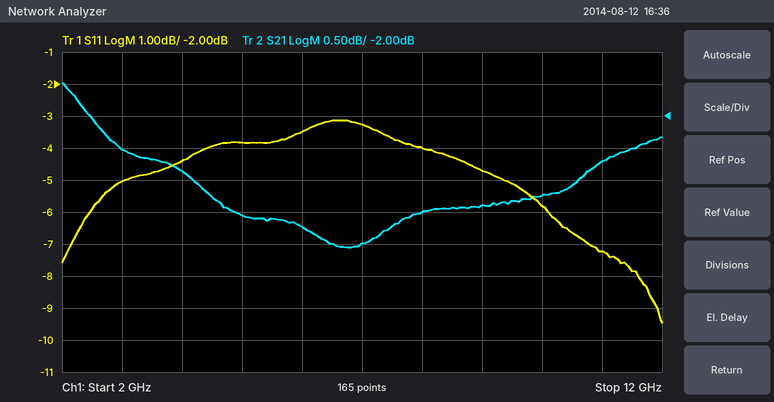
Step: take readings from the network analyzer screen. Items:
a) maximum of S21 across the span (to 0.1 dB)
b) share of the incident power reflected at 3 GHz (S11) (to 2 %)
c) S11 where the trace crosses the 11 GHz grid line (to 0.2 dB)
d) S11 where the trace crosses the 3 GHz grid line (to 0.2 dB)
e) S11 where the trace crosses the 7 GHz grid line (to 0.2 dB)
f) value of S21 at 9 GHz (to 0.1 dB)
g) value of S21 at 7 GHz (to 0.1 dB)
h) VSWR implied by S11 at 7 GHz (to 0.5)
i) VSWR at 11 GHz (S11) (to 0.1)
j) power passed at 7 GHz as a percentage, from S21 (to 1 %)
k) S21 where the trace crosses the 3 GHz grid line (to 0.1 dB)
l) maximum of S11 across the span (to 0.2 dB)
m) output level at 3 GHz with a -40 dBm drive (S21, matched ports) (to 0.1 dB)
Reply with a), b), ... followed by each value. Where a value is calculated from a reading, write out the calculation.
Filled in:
a) -1.5 dB
b) 10^(-5/10) ≈ 32 %
c) -7.2 dB
d) -5.0 dB
e) -3.2 dB
f) -3.4 dB
g) -4.0 dB
h) |Γ| = 10^(-3.2/20) = 0.6918; VSWR = (1 + 0.6918)/(1 − 0.6918) ≈ 5.5
i) |Γ| = 10^(-7.2/20) = 0.4365; VSWR = (1 + 0.4365)/(1 − 0.4365) ≈ 2.5
j) 10^(-4/10) ≈ 40 %
k) -2.5 dB
l) -3.2 dB
m) -40 dBm + (-2.5 dB) = -42.5 dBm
